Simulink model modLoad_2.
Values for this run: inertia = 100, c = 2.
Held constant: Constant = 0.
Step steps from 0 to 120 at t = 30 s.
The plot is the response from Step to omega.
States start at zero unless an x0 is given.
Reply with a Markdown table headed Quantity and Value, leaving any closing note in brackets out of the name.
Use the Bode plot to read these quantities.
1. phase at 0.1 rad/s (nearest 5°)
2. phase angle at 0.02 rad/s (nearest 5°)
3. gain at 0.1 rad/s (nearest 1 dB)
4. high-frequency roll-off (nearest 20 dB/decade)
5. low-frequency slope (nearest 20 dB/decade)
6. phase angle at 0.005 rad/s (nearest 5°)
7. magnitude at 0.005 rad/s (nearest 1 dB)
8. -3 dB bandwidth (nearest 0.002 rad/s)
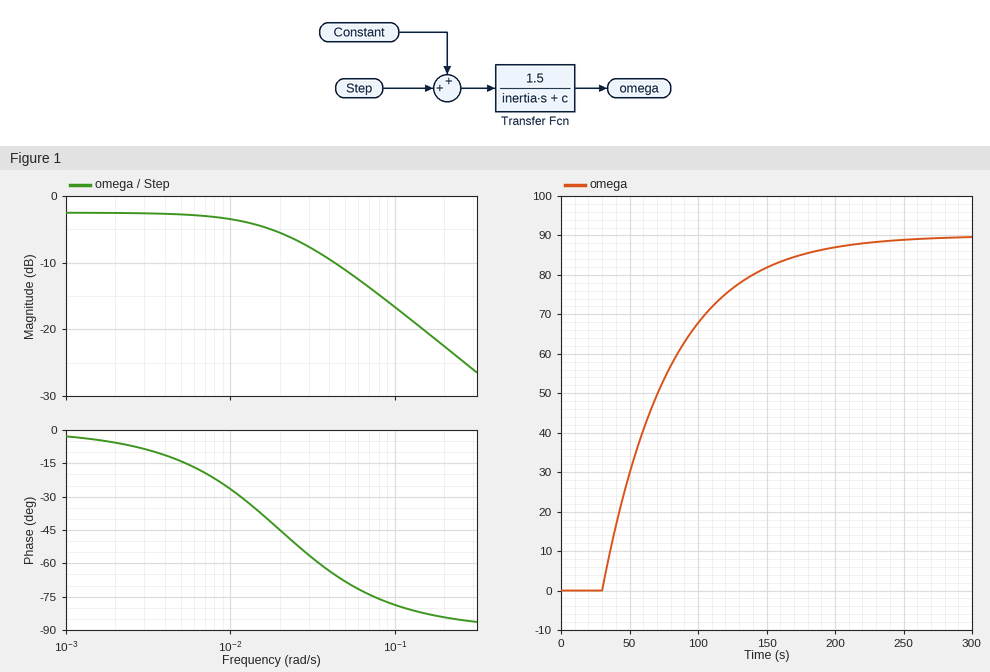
| Quantity | Value |
|---|---|
| phase at 0.1 rad/s | -80° |
| phase angle at 0.02 rad/s | -45° |
| gain at 0.1 rad/s | -17 dB |
| high-frequency roll-off | -20 dB/decade |
| low-frequency slope | 0 dB/decade |
| phase angle at 0.005 rad/s | -15° |
| magnitude at 0.005 rad/s | -3 dB |
| -3 dB bandwidth | 0.020 rad/s |
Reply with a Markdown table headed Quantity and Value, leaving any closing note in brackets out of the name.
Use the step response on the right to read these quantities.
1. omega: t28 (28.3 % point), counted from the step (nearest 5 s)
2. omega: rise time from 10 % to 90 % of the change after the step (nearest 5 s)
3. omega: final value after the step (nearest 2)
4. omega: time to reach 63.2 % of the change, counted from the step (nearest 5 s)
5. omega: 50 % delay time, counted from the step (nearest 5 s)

| Quantity | Value |
|---|---|
| omega: t28 (28.3 % point), counted from the step | 15 s |
| omega: rise time from 10 % to 90 % of the change after the step | 110 s |
| omega: final value after the step | 90 |
| omega: time to reach 63.2 % of the change, counted from the step | 50 s |
| omega: 50 % delay time, counted from the step | 35 s |
